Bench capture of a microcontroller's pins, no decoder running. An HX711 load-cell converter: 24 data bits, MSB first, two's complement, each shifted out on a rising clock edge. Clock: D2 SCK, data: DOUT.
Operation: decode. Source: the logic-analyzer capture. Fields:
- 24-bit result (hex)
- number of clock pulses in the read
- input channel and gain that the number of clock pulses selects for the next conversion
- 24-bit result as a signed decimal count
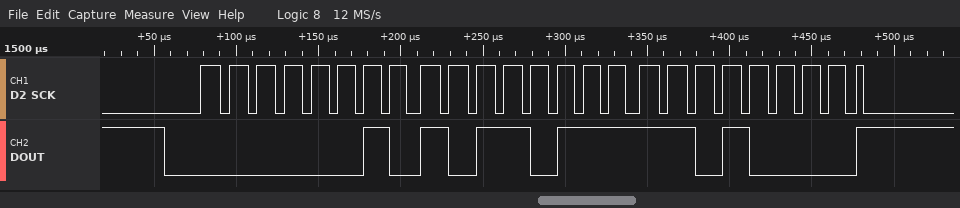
0x02B7D0
25
channel A, gain 128
178128
